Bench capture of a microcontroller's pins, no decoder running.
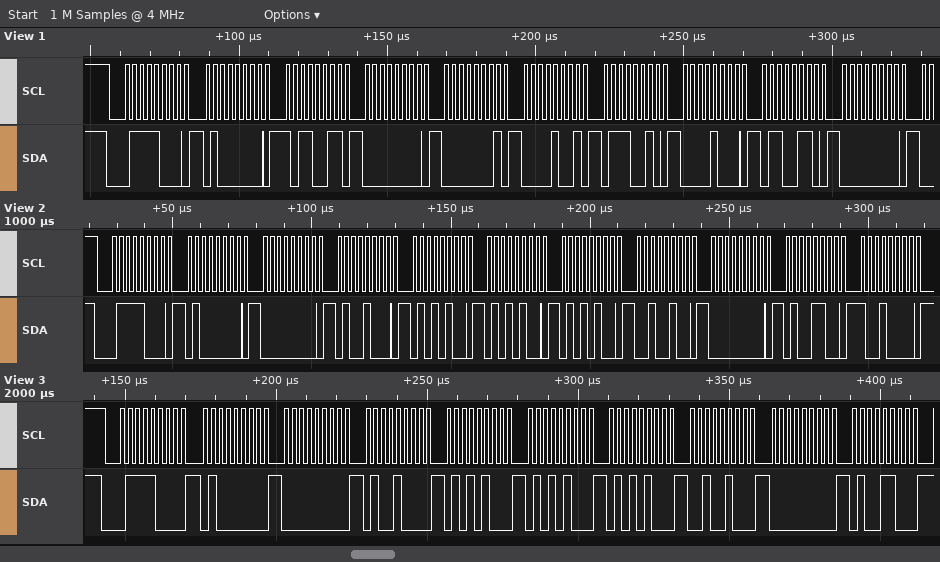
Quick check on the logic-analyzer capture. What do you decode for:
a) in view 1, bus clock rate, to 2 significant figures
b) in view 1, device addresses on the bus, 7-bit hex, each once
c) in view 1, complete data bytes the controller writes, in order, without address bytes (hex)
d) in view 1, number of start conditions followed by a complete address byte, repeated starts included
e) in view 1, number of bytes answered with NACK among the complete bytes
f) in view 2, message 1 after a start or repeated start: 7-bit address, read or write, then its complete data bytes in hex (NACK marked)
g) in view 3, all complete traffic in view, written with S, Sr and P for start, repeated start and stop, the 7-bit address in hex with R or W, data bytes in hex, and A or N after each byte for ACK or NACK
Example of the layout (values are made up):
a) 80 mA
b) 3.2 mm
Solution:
a) 400 kHz
b) 0x3C
c) 40 B3 00 01 09 72 08 66 00
d) 1
e) 0
f) 0x3C write: 40 00 48 54 54 54 24 00 4C 90
g) S 3CW A 40 A 00 A 48 A 54 A 54 A 54 A 24 A 00 A 4C A
